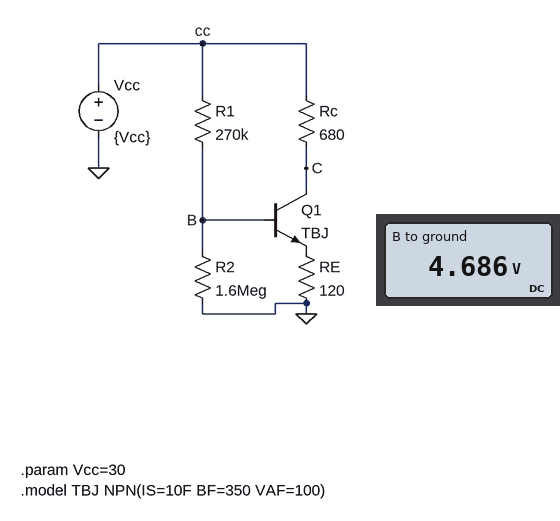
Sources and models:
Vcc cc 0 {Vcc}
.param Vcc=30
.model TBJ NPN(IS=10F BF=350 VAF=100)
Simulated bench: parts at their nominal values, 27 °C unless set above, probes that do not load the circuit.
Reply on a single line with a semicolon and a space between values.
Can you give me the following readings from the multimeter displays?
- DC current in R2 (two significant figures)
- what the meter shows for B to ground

2.9 µA; 4.686 V
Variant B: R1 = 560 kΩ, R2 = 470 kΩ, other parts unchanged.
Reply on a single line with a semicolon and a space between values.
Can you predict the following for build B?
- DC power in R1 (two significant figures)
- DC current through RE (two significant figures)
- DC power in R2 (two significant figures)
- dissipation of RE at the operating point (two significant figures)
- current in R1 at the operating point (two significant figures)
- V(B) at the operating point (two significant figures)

1.3 mW; 17 mA; 17 µW; 36 mW; 49 µA; 2.8 V
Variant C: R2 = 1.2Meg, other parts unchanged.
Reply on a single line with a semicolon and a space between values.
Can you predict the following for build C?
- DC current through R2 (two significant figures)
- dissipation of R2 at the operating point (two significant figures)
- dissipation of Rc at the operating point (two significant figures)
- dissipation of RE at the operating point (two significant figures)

3.9 µA; 18 µW; 720 mW; 130 mW
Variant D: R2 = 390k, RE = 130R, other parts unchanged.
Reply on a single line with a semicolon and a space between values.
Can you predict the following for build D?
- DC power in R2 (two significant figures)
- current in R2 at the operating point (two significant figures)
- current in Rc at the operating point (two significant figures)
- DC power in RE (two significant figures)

56 µW; 12 µA; 30 mA; 120 mW
